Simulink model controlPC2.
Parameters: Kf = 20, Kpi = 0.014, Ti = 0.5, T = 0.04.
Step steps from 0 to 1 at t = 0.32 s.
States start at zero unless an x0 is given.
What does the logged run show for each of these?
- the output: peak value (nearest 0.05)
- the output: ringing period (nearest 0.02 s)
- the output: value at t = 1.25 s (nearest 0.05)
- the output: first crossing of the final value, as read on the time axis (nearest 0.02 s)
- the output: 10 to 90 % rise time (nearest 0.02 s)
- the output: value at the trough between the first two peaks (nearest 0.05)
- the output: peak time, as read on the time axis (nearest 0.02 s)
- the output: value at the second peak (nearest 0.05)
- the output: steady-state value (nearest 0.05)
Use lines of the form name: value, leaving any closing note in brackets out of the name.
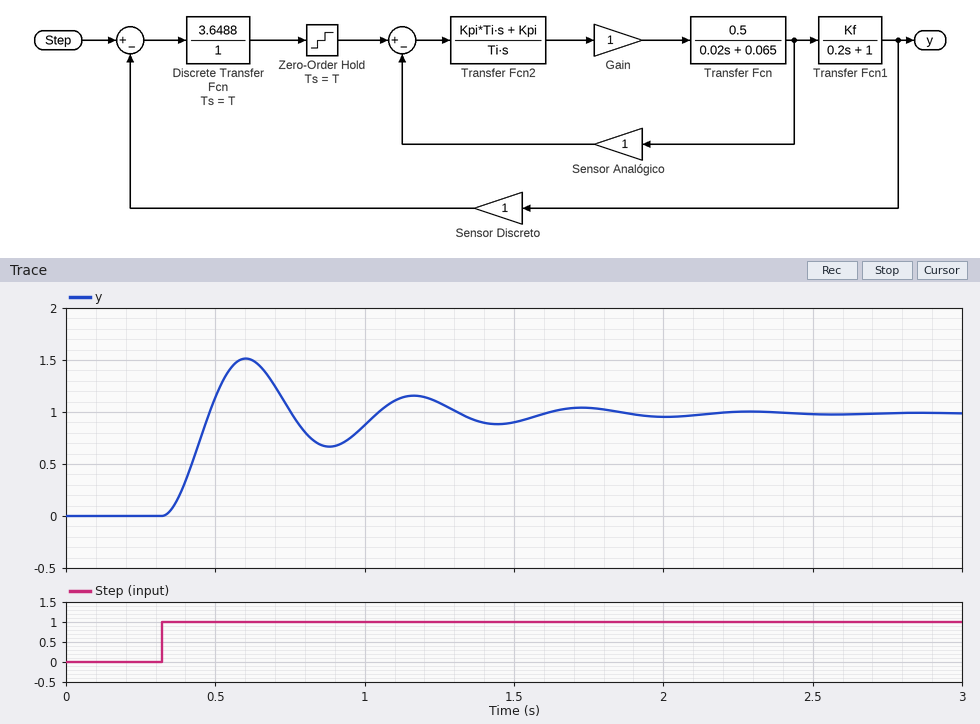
the output: peak value: 1.50
the output: ringing period: 0.56 s
the output: value at t = 1.25 s: 1.10
the output: first crossing of the final value, as read on the time axis: 0.48 s
the output: 10 to 90 % rise time: 0.10 s
the output: value at the trough between the first two peaks: 0.65
the output: peak time, as read on the time axis: 0.60 s
the output: value at the second peak: 1.15
the output: steady-state value: 1.00
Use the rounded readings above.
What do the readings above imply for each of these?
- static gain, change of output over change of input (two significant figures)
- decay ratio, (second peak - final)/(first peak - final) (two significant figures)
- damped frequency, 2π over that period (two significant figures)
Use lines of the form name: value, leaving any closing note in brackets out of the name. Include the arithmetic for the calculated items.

static gain, change of output over change of input: (1 - 0) / (1 - 0) = 1.0
decay ratio, (second peak - final)/(first peak - final): (1.15 - 1) / (1.5 - 1) = 0.30
damped frequency, 2π over that period: 2π / 0.56 = 11 rad/s
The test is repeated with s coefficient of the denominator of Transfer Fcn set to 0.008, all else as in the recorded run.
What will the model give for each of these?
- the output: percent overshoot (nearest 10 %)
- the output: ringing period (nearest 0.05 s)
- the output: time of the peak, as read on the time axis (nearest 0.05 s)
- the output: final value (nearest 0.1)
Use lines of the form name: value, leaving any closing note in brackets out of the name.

the output: percent overshoot: 50 %
the output: ringing period: 0.35 s
the output: time of the peak, as read on the time axis: 0.50 s
the output: final value: 1.0
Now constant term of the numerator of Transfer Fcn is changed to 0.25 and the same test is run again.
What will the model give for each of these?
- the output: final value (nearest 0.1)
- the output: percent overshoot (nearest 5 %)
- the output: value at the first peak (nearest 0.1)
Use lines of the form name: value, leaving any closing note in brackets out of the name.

the output: final value: 1.0
the output: percent overshoot: 30 %
the output: value at the first peak: 1.3
